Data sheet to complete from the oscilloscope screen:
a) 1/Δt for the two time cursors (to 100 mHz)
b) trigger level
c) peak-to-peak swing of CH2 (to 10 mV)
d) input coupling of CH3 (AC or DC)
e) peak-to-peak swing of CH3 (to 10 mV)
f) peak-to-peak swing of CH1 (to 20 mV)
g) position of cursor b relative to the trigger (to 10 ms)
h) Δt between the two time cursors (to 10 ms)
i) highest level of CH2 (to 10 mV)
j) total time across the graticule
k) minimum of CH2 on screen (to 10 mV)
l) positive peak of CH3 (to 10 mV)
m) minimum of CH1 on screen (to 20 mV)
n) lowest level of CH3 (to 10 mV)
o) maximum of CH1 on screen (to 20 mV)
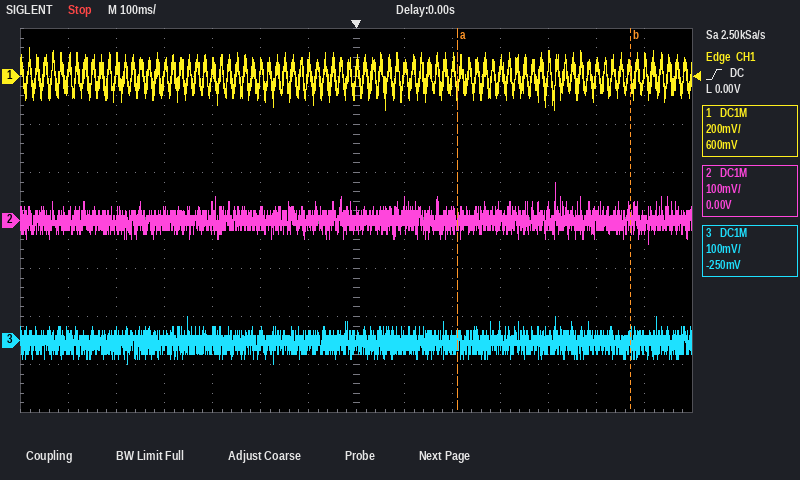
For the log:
2.8 Hz
0.00 V
130 mV
DC
100 mV
260 mV
+570 ms
360 ms
80 mV
1.4 s
-50 mV
50 mV
-140 mV
-50 mV
120 mV
